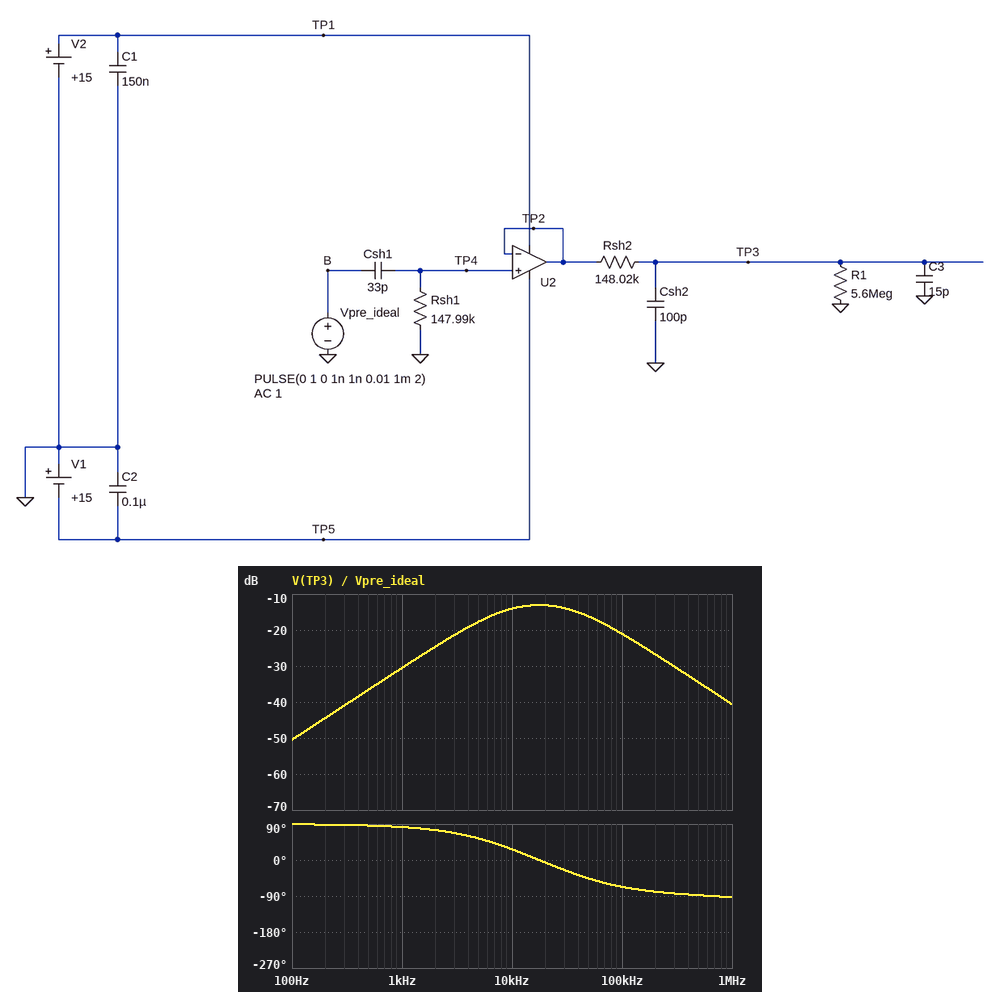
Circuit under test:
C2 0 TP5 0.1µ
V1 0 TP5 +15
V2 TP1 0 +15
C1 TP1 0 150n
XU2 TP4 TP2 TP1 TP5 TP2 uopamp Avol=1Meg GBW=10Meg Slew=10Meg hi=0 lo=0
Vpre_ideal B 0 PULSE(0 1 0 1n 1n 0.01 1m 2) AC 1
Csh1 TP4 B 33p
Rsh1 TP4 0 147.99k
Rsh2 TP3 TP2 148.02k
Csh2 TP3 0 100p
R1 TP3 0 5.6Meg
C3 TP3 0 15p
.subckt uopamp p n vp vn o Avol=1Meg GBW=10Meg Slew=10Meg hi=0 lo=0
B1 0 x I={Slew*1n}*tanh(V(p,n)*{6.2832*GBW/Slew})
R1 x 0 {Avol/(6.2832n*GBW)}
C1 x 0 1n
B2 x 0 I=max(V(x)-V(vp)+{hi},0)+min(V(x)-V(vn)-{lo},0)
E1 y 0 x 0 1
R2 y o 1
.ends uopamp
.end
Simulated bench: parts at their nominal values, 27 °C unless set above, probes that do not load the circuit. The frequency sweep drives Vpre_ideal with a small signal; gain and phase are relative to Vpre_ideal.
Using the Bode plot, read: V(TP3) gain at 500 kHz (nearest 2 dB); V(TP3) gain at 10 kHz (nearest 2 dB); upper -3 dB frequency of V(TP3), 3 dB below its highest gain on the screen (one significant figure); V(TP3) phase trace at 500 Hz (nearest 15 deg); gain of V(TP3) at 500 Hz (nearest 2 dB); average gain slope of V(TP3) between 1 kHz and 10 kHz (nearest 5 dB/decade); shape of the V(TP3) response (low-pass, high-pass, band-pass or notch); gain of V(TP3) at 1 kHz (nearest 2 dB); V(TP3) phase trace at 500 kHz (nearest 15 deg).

-34 dB
-14 dB
50 kHz
90 deg
-36 dB
15 dB/decade
band-pass
-30 dB
-90 deg
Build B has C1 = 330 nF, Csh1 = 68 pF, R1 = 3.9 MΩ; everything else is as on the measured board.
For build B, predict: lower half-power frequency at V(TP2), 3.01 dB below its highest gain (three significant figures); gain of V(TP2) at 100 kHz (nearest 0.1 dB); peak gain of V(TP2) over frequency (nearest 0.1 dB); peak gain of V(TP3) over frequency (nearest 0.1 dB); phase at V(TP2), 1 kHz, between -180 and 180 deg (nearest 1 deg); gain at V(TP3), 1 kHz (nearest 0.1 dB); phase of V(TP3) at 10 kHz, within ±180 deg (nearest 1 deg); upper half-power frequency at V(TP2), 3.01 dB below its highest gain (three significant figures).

15.8 kHz
-0.1 dB
0 dB
-8.7 dB
86 deg
-24.4 dB
12 deg
10.0 MHz
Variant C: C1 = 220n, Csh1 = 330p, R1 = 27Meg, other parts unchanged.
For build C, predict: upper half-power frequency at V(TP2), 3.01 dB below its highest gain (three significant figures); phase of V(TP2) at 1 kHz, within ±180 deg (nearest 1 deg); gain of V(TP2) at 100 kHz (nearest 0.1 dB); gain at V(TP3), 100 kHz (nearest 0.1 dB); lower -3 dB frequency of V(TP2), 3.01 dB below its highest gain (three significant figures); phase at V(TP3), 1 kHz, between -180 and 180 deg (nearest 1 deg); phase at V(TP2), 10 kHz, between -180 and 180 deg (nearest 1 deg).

10.0 MHz
73 deg
0 dB
-20.6 dB
3.26 kHz
67 deg
18 deg
